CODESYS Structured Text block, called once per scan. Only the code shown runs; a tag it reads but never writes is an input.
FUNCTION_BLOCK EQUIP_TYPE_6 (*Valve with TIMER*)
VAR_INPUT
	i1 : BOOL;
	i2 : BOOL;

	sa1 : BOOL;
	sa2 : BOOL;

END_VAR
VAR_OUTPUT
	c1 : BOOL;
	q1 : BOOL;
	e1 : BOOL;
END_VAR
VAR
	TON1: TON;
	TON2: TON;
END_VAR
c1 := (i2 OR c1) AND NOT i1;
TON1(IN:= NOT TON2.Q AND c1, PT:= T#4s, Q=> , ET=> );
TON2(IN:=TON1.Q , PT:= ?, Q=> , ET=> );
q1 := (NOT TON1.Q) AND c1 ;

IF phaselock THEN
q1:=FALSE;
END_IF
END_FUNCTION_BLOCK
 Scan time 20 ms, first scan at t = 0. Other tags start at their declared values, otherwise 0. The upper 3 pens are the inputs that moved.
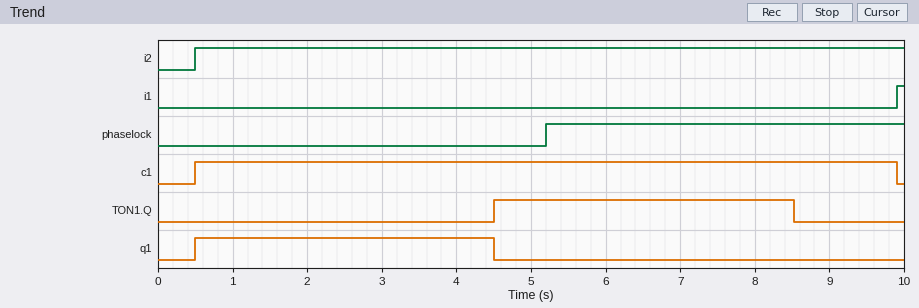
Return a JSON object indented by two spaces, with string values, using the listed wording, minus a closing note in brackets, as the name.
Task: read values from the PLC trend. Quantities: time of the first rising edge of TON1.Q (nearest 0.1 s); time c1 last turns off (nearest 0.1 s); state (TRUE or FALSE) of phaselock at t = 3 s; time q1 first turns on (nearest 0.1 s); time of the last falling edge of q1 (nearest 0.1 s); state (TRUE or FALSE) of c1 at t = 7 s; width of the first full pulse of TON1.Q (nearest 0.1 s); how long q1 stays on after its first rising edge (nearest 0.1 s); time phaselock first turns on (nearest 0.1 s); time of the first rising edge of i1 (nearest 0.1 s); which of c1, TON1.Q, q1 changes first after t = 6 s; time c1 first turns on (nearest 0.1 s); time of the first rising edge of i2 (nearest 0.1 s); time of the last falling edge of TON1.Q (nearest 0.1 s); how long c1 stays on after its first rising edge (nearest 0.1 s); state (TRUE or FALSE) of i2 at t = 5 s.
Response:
{
  "time of the first rising edge of TON1.Q": "4.5 s",
  "time c1 last turns off": "9.9 s",
  "state (TRUE or FALSE) of phaselock at t = 3 s": "FALSE",
  "time q1 first turns on": "0.5 s",
  "time of the last falling edge of q1": "4.5 s",
  "state (TRUE or FALSE) of c1 at t = 7 s": "TRUE",
  "width of the first full pulse of TON1.Q": "4.0 s",
  "how long q1 stays on after its first rising edge": "4.0 s",
  "time phaselock first turns on": "5.2 s",
  "time of the first rising edge of i1": "9.9 s",
  "which of c1, TON1.Q, q1 changes first after t = 6 s": "TON1.Q",
  "time c1 first turns on": "0.5 s",
  "time of the first rising edge of i2": "0.5 s",
  "time of the last falling edge of TON1.Q": "8.5 s",
  "how long c1 stays on after its first rising edge": "9.4 s",
  "state (TRUE or FALSE) of i2 at t = 5 s": "TRUE"
}
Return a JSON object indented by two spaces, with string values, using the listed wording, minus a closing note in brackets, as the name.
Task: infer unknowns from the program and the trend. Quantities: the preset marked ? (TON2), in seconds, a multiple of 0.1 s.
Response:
{
  "the preset marked ? (TON2), in seconds, a multiple of 0.1 s": "4.0 s"
}
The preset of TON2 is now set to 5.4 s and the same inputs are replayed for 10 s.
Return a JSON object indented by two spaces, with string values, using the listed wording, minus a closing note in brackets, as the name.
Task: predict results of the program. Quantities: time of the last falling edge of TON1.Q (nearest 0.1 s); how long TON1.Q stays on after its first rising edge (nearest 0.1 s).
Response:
{
  "time of the last falling edge of TON1.Q": "9.9 s",
  "how long TON1.Q stays on after its first rising edge": "5.4 s"
}
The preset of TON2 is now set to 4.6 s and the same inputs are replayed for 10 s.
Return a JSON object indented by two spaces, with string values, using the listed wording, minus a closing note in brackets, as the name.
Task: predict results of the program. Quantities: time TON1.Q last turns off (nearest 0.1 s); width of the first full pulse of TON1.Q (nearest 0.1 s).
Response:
{
  "time TON1.Q last turns off": "9.1 s",
  "width of the first full pulse of TON1.Q": "4.6 s"
}
